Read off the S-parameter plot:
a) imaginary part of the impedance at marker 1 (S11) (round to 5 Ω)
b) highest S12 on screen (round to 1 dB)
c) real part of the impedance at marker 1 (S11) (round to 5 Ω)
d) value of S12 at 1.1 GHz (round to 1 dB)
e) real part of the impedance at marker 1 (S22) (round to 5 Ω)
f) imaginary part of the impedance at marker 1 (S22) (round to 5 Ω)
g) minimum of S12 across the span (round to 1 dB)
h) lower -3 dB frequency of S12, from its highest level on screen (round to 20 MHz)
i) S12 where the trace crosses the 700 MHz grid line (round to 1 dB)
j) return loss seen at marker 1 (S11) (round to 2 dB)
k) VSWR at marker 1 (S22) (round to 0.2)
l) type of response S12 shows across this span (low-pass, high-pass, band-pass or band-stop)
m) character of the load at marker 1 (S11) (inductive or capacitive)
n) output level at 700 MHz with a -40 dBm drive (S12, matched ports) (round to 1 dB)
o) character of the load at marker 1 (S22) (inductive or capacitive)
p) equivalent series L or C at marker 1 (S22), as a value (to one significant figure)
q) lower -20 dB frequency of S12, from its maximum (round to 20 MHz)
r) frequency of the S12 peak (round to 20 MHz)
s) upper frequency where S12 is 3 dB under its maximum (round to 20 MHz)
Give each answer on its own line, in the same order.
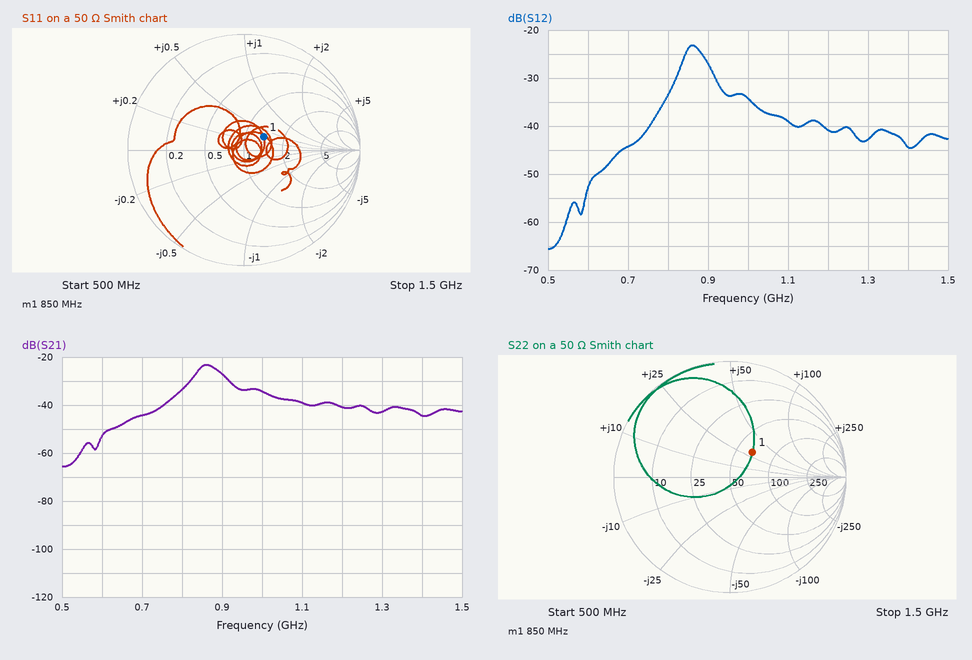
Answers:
+15 Ω
-23 dB
70 Ω
-39 dB
65 Ω
+30 Ω
-66 dB
840 MHz
-44 dB
14 dB
1.8
band-pass
inductive
-84 dBm
inductive
6 nH
720 MHz
860 MHz
900 MHz
